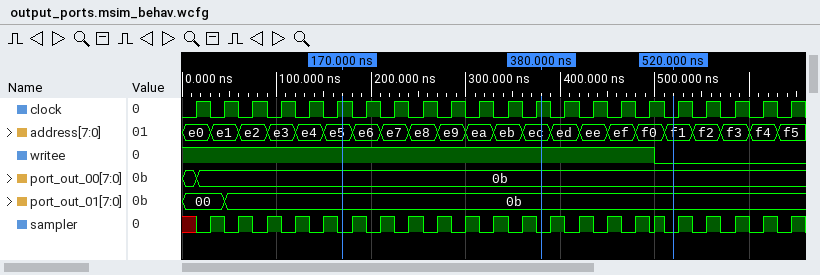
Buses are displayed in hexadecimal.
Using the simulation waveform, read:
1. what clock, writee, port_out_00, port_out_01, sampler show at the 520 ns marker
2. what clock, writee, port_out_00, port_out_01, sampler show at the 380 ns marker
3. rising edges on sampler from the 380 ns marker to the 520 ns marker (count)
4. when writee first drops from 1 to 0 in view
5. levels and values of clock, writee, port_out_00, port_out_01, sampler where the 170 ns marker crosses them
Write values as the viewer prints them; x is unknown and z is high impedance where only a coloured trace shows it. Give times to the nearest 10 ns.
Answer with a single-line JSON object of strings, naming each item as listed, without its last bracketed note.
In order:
{"what clock, writee, port_out_00, port_out_01, sampler show at the 520 ns marker": "clock=0, writee=0, port_out_00=0b, port_out_01=0b, sampler=0", "what clock, writee, port_out_00, port_out_01, sampler show at the 380 ns marker": "clock=1, writee=1, port_out_00=0b, port_out_01=0b, sampler=0", "rising edges on sampler from the 380 ns marker to the 520 ns marker": "5", "when writee first drops from 1 to 0 in view": "500 ns", "levels and values of clock, writee, port_out_00, port_out_01, sampler where the 170 ns marker crosses them": "clock=1, writee=1, port_out_00=0b, port_out_01=0b, sampler=0"}
